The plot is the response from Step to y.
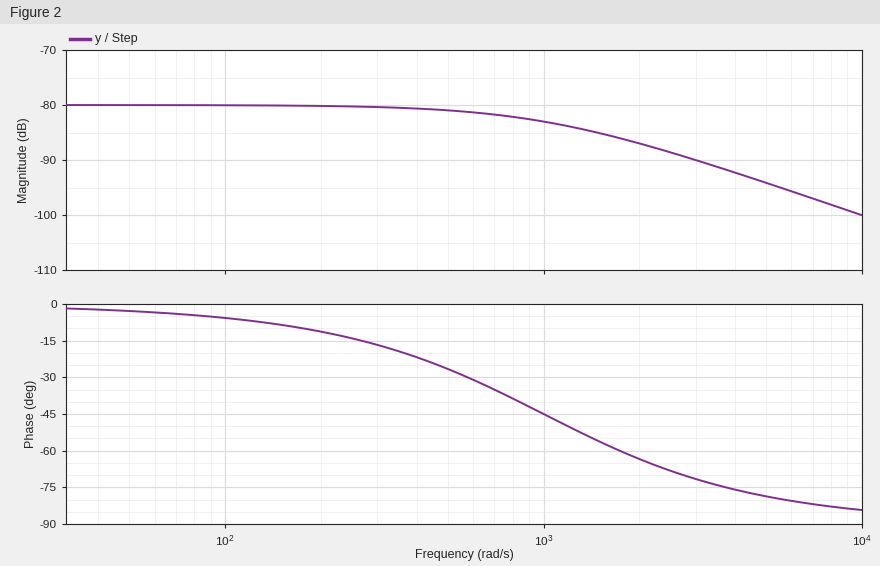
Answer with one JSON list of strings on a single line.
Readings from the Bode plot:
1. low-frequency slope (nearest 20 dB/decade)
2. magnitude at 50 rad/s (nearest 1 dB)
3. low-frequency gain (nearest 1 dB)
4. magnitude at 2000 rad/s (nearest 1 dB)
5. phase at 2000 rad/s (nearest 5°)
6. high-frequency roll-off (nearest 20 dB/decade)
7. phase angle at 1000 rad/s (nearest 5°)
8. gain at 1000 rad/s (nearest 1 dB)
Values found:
["0 dB/decade", "-80 dB", "-80 dB", "-87 dB", "-65°", "-20 dB/decade", "-45°", "-83 dB"]
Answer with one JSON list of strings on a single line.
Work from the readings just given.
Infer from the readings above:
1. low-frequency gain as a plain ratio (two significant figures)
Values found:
["0.00010"]
